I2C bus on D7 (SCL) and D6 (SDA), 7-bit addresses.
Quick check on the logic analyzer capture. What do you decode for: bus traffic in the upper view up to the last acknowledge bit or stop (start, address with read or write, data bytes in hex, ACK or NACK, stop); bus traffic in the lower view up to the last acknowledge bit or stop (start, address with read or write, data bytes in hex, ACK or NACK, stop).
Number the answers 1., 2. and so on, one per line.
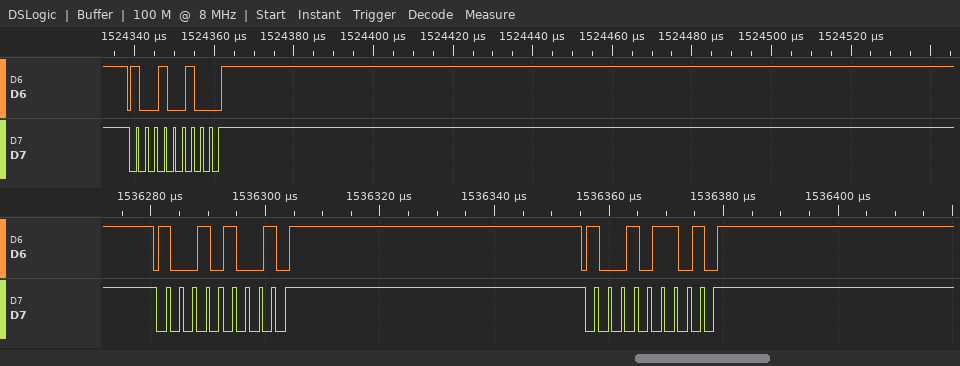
1. start, address 49 write ACK, stop
2. start, address 4A write NACK, stop, start, address 4B write NACK, stop
